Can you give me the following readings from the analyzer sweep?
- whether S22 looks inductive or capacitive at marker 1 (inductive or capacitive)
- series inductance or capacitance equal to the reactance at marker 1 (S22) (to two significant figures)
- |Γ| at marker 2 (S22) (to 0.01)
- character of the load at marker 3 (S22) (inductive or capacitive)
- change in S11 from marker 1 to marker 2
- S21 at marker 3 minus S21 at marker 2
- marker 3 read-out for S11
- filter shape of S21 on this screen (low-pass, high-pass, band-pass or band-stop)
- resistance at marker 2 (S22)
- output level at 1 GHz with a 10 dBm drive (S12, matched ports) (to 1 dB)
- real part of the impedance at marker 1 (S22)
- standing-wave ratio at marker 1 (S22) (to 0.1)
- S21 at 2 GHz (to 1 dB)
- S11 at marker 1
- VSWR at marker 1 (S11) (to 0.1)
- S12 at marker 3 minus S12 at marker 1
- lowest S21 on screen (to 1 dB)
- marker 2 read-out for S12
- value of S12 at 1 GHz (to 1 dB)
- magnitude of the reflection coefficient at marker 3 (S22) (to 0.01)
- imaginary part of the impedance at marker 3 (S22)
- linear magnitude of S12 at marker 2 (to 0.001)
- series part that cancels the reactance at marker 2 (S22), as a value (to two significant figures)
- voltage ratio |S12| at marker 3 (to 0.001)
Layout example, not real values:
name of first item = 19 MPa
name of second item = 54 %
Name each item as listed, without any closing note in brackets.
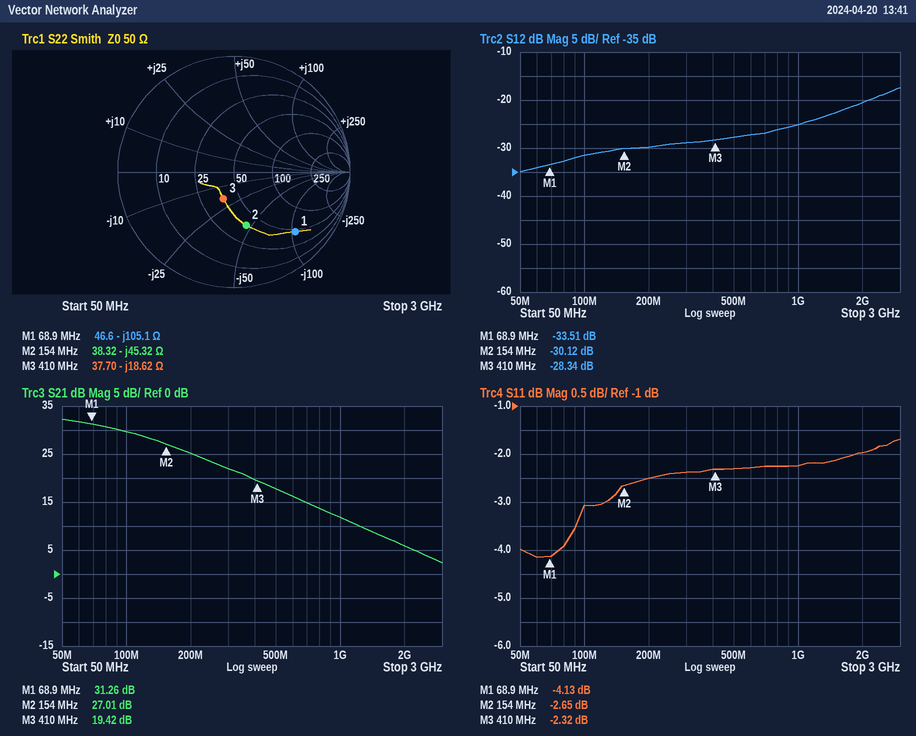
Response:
whether S22 looks inductive or capacitive at marker 1 = capacitive
series inductance or capacitance equal to the reactance at marker 1 (S22) = 22 pF
|Γ| at marker 2 (S22) = 0.47
character of the load at marker 3 (S22) = capacitive
change in S11 from marker 1 to marker 2 = 1.48 dB
S21 at marker 3 minus S21 at marker 2 = -7.59 dB
marker 3 read-out for S11 = -2.32 dB
filter shape of S21 on this screen = low-pass
resistance at marker 2 = 38.32 Ω
output level at 1 GHz with a 10 dBm drive (S12, matched ports) = -15 dBm
real part of the impedance at marker 1 = 46.6 Ω
standing-wave ratio at marker 1 (S22) = 6.6
S21 at 2 GHz = 6 dB
S11 at marker 1 = -4.13 dB
VSWR at marker 1 (S11) = 4.3
S12 at marker 3 minus S12 at marker 1 = 5.17 dB
lowest S21 on screen = 2 dB
marker 2 read-out for S12 = -30.12 dB
value of S12 at 1 GHz = -25 dB
magnitude of the reflection coefficient at marker 3 (S22) = 0.25
imaginary part of the impedance at marker 3 = -18.62 Ω
linear magnitude of S12 at marker 2 = 0.031
series part that cancels the reactance at marker 2 (S22), as a value = 47 nH
voltage ratio |S12| at marker 3 = 0.038
